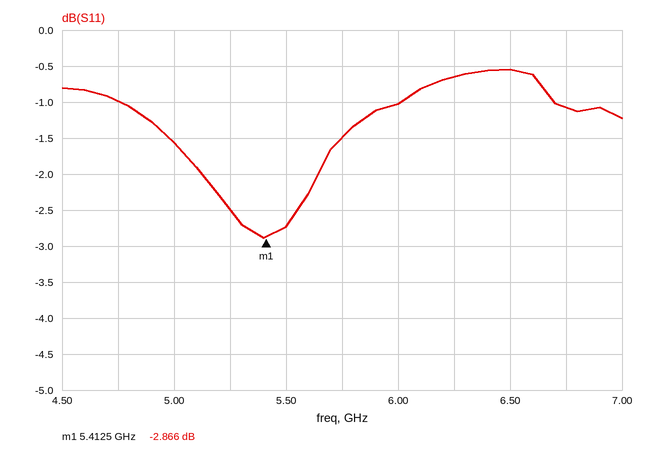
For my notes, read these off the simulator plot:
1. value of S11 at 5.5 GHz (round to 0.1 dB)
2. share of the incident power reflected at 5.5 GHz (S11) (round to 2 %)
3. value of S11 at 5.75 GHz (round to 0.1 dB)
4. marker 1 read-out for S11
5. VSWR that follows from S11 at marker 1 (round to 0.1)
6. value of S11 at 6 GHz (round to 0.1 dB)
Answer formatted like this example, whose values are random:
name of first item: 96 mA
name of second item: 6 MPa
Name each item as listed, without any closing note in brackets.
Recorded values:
value of S11 at 5.5 GHz: -2.7 dB
share of the incident power reflected at 5.5 GHz (S11): 54 %
value of S11 at 5.75 GHz: -1.5 dB
marker 1 read-out for S11: -2.866 dB
VSWR that follows from S11 at marker 1: 6.1
value of S11 at 6 GHz: -1.0 dB
